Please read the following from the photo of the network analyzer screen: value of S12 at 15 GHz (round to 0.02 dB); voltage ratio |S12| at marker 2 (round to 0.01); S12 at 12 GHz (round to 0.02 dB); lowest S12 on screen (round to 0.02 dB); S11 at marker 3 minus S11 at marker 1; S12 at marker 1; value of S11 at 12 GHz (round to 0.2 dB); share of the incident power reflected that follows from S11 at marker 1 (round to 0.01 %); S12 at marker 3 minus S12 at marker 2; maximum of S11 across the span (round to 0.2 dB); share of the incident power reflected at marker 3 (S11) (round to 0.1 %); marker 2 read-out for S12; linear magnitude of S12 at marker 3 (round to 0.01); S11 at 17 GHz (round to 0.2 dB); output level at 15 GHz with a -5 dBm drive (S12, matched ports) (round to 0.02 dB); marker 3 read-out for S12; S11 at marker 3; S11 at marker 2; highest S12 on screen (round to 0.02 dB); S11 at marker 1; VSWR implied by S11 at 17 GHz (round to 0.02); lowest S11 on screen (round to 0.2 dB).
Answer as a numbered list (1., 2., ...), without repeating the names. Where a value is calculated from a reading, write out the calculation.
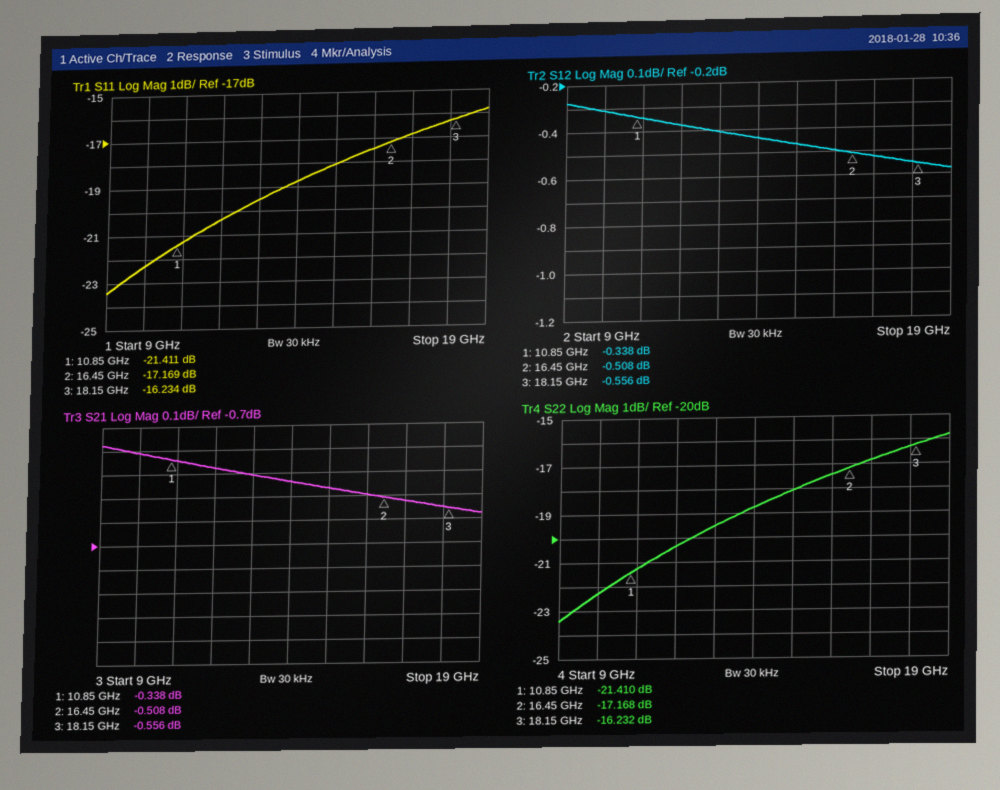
1. -0.46 dB
2. 10^(-0.508/20) ≈ 0.94
3. -0.38 dB
4. -0.58 dB
5. -16.234 − (-21.411) = 5.177 dB
6. -0.338 dB
7. -20.4 dB
8. 10^(-21.411/10) ≈ 0.72 %
9. -0.556 − (-0.508) = -0.048 dB
10. -15.8 dB
11. 10^(-16.234/10) ≈ 2.4 %
12. -0.508 dB
13. 10^(-0.556/20) ≈ 0.94
14. -16.8 dB
15. -5 dBm + (-0.46 dB) = -5.46 dBm
16. -0.556 dB
17. -16.234 dB
18. -17.169 dB
19. -0.28 dB
20. -21.411 dB
21. |Γ| = 10^(-16.8/20) = 0.1445; VSWR = (1 + 0.1445)/(1 − 0.1445) ≈ 1.34
22. -23.4 dB
